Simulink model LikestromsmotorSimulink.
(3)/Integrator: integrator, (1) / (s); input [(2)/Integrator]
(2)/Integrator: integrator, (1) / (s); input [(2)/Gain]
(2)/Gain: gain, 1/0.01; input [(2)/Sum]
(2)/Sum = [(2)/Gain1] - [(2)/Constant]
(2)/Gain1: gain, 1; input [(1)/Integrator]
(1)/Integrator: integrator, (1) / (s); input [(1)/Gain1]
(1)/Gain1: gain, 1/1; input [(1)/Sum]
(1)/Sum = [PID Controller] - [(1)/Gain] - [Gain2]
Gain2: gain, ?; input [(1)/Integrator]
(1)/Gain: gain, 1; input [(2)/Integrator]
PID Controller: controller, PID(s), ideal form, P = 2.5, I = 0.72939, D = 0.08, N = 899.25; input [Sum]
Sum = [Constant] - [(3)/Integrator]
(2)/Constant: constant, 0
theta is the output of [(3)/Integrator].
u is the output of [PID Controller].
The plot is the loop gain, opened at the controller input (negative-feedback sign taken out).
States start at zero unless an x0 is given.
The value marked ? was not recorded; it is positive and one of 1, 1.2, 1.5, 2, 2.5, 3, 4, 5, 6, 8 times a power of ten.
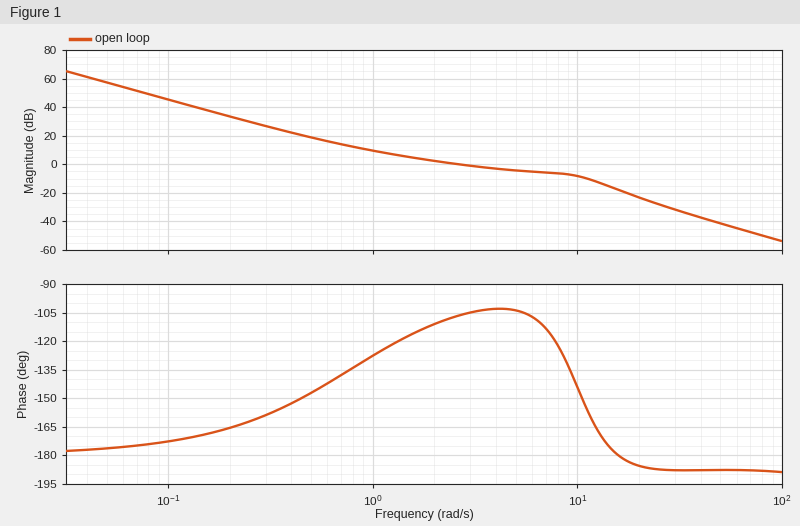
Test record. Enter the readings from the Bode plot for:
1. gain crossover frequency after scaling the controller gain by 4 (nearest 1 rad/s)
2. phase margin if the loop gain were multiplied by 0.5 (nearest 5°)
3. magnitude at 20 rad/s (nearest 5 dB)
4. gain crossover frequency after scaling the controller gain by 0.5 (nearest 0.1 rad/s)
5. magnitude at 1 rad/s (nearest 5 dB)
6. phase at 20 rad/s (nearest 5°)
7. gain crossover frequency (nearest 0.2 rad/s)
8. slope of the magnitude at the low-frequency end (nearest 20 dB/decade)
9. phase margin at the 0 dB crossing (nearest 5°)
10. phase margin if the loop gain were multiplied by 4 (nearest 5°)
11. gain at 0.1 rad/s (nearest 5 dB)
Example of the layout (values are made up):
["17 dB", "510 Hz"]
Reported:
["12 rad/s", "60°", "-25 dB", "1.4 rad/s", "10 dB", "-185°", "2.6 rad/s", "-40 dB/decade", "75°", "15°", "45 dB"]
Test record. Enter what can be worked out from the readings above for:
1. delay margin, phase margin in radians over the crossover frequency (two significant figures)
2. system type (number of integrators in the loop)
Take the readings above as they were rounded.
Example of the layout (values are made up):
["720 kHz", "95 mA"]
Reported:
["0.50 s", "2"]
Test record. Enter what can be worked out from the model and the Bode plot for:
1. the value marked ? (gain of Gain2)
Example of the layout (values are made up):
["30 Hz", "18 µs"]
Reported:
["8"]
